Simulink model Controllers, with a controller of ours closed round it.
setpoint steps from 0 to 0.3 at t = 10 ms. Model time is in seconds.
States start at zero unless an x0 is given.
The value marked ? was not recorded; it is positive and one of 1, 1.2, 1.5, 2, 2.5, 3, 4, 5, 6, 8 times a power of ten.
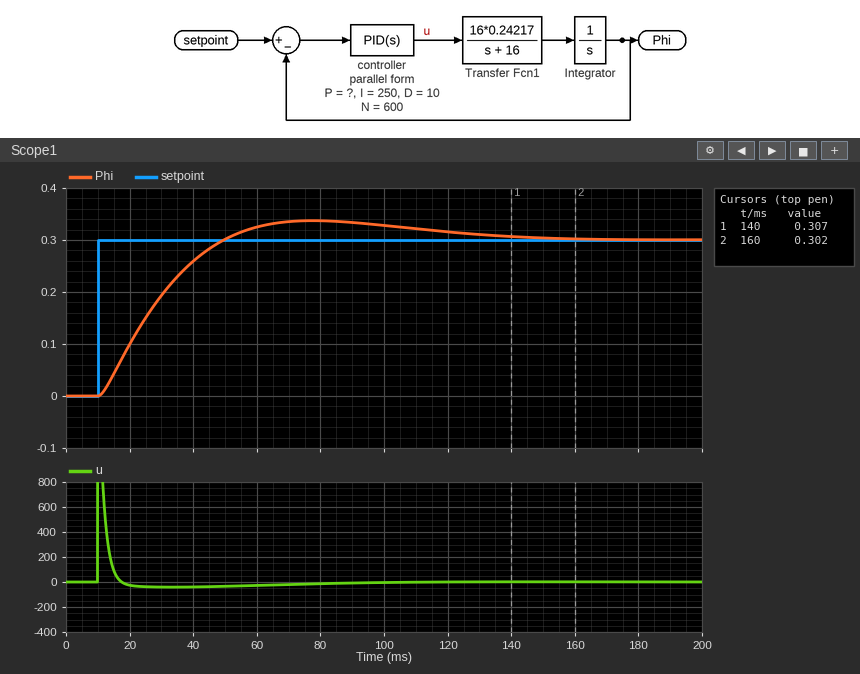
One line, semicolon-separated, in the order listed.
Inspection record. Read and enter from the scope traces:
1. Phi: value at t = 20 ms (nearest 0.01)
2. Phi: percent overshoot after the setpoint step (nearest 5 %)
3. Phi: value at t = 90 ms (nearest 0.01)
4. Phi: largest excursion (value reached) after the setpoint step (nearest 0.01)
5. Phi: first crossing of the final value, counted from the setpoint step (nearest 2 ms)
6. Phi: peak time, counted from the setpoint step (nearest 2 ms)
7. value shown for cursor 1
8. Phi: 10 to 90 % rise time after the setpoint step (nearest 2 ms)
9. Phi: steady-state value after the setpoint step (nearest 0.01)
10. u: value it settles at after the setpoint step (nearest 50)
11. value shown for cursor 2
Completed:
0.10; 10 %; 0.33; 0.34; 40 ms; 68 ms; 0.307; 28 ms; 0.30; 0; 0.302
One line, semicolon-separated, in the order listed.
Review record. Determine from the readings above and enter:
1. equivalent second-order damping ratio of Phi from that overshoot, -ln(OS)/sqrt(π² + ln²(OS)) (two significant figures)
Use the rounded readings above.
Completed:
0.59
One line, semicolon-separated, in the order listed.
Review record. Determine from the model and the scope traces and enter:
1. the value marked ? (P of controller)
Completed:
400
